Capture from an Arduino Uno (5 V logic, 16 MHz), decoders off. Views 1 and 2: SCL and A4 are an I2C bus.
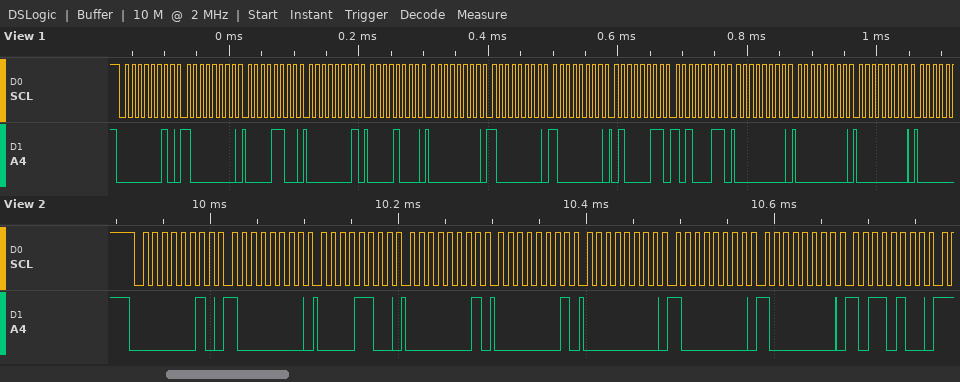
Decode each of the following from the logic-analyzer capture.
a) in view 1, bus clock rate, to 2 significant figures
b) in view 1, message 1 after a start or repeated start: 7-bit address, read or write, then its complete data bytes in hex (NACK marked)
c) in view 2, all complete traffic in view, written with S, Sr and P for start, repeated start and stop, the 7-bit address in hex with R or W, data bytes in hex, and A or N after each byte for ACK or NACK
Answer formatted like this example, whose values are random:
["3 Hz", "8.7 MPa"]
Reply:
["100 kHz", "0x01 write: 80 0C 01 08 00 80 80 43 A3 00 00 00", "S 01W A 80 A 0C A 01 A 01 A 00 A 80 A 80 A B4 A"]
